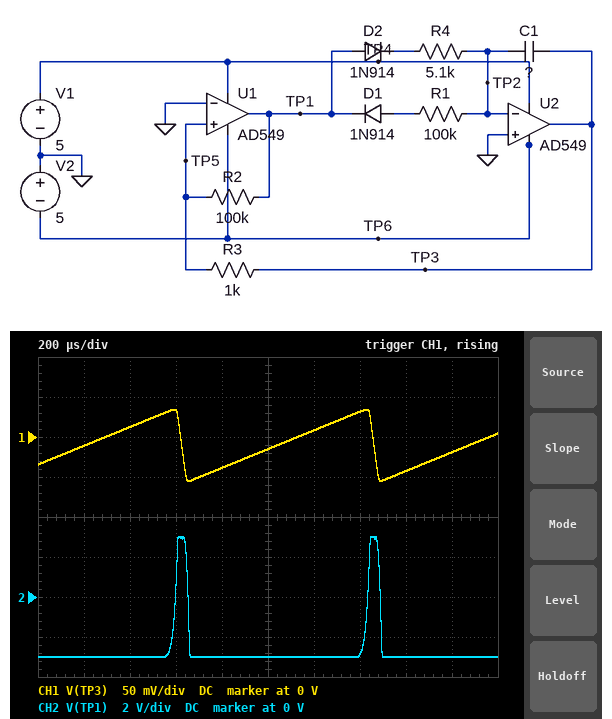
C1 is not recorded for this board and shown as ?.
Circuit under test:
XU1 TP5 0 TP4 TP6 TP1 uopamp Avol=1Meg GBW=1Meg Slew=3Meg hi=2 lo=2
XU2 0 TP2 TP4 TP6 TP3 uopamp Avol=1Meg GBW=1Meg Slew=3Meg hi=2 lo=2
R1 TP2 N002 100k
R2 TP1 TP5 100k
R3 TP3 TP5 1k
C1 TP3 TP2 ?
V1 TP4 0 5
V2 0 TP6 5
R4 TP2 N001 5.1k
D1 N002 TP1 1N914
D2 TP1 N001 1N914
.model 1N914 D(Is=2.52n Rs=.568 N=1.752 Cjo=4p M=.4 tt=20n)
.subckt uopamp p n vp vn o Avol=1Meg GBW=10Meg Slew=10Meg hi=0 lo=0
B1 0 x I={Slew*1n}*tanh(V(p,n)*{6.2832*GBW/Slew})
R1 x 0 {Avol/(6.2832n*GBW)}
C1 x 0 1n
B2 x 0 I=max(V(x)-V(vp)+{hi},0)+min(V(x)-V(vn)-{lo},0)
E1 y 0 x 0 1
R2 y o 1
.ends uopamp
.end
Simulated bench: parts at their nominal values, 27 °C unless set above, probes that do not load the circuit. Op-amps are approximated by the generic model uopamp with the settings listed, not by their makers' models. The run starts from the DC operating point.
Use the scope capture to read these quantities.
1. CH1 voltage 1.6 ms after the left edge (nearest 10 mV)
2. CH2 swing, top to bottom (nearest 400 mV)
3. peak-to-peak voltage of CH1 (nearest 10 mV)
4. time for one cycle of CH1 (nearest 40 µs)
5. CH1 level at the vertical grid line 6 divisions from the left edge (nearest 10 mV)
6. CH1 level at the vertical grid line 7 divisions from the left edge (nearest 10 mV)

-40 mV
6.0 V
90 mV
840 µs
10 mV
30 mV
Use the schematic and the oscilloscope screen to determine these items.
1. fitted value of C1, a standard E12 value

220 nF
